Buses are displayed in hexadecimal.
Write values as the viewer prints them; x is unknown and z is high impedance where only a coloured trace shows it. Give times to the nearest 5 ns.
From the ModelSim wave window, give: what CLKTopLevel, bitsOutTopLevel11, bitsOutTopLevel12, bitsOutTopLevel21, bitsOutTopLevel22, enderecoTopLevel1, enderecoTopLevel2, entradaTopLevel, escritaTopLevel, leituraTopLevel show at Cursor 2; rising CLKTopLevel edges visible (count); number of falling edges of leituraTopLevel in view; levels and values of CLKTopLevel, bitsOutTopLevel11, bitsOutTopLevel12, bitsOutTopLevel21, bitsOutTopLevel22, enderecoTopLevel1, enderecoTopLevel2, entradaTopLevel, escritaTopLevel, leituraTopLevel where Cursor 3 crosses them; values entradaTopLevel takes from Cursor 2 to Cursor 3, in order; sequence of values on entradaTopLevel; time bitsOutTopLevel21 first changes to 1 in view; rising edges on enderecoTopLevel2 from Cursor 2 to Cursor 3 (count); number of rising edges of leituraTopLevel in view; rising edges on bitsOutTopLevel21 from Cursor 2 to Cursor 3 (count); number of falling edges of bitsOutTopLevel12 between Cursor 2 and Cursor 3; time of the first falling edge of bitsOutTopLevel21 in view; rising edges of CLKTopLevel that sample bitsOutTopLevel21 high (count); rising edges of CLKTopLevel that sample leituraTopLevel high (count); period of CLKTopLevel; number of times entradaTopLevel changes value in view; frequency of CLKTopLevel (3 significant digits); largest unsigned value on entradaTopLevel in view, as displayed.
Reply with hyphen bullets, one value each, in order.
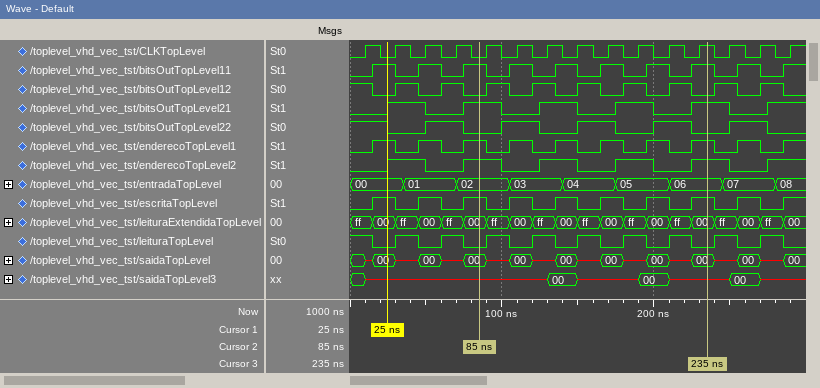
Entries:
- CLKTopLevel=0, bitsOutTopLevel11=1, bitsOutTopLevel12=0, bitsOutTopLevel21=1, bitsOutTopLevel22=0, enderecoTopLevel1=1, enderecoTopLevel2=1, entradaTopLevel=02, escritaTopLevel=1, leituraTopLevel=0
- 15
- 10
- CLKTopLevel=1, bitsOutTopLevel11=1, bitsOutTopLevel12=0, bitsOutTopLevel21=1, bitsOutTopLevel22=0, enderecoTopLevel1=1, enderecoTopLevel2=1, entradaTopLevel=06, escritaTopLevel=1, leituraTopLevel=0
- 02, 03, 04, 05, 06
- 00, 01, 02, 03, 04, 05, 06, 07, 08
- 25 ns
- 3
- 9
- 3
- 5
- 50 ns
- 9
- 5
- 20 ns
- 8
- 50.0 MHz
- 08
